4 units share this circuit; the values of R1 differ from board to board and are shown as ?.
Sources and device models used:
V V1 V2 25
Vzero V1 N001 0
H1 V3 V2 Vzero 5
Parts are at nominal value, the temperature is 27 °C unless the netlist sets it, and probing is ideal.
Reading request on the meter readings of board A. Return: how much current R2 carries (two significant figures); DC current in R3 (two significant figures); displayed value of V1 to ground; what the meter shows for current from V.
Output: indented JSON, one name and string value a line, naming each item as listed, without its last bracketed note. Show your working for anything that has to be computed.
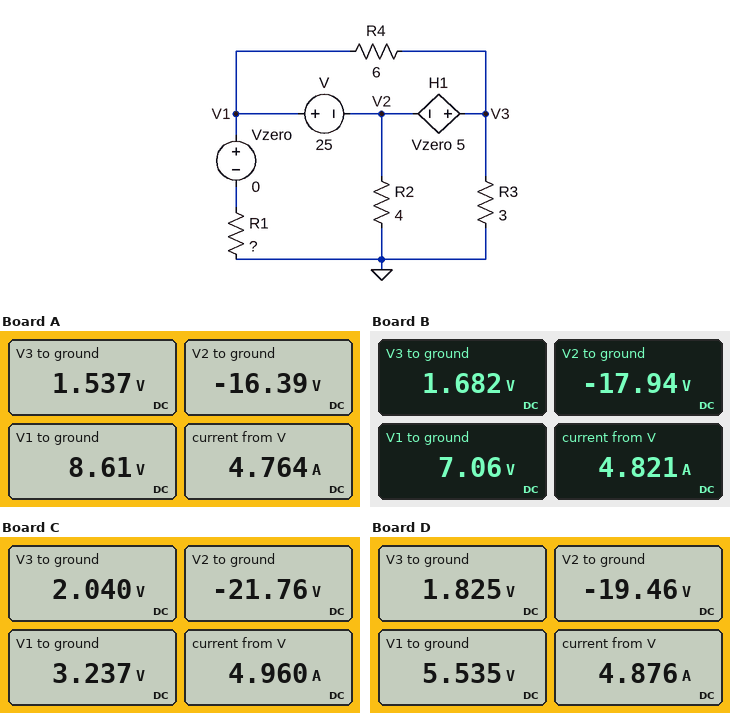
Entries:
{
  "how much current R2 carries": "(0 V - (-16.39 V)) / 4 Ω = 4.1 A",
  "DC current in R3": "(1.537 V) / 3 Ω = 510 mA",
  "displayed value of V1 to ground": "8.61 V",
  "what the meter shows for current from V": "4.764 A"
}
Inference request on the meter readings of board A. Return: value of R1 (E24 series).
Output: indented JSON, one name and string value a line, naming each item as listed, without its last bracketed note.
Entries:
{
  "value of R1": "2.4 Ω"
}
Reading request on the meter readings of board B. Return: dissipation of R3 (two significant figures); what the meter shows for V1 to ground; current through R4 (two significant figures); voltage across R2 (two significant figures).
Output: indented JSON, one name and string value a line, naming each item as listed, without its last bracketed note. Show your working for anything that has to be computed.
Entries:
{
  "dissipation of R3": "(1.682 V)^2 / 3 Ω = 940 mW",
  "what the meter shows for V1 to ground": "7.06 V",
  "current through R4": "(7.06 V - 1.682 V) / 6 Ω = 900 mA",
  "voltage across R2": "0 V - (-17.94 V) = 18 V"
}
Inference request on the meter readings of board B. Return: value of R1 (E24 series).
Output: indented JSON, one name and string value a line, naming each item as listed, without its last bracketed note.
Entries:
{
  "value of R1": "1.8 Ω"
}
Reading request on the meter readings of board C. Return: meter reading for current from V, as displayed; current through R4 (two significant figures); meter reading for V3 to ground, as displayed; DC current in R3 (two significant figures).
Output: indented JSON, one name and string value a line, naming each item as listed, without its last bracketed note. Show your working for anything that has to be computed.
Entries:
{
  "meter reading for current from V, as displayed": "4.960 A",
  "current through R4": "(3.237 V - 2.04 V) / 6 Ω = 200 mA",
  "meter reading for V3 to ground, as displayed": "2.040 V",
  "DC current in R3": "(2.04 V) / 3 Ω = 680 mA"
}
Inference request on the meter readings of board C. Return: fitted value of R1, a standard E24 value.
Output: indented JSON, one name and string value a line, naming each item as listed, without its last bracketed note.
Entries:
{
  "fitted value of R1, a standard E24 value": "0.68 Ω"
}
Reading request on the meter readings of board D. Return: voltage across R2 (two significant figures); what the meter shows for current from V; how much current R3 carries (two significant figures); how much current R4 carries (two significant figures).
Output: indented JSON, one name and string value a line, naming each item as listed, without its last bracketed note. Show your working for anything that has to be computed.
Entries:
{
  "voltage across R2": "0 V - (-19.46 V) = 19 V",
  "what the meter shows for current from V": "4.876 A",
  "how much current R3 carries": "(1.825 V) / 3 Ω = 610 mA",
  "how much current R4 carries": "(5.535 V - 1.825 V) / 6 Ω = 620 mA"
}
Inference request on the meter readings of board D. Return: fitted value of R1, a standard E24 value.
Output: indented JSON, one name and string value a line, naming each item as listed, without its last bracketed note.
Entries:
{
  "fitted value of R1, a standard E24 value": "1.3 Ω"
}
